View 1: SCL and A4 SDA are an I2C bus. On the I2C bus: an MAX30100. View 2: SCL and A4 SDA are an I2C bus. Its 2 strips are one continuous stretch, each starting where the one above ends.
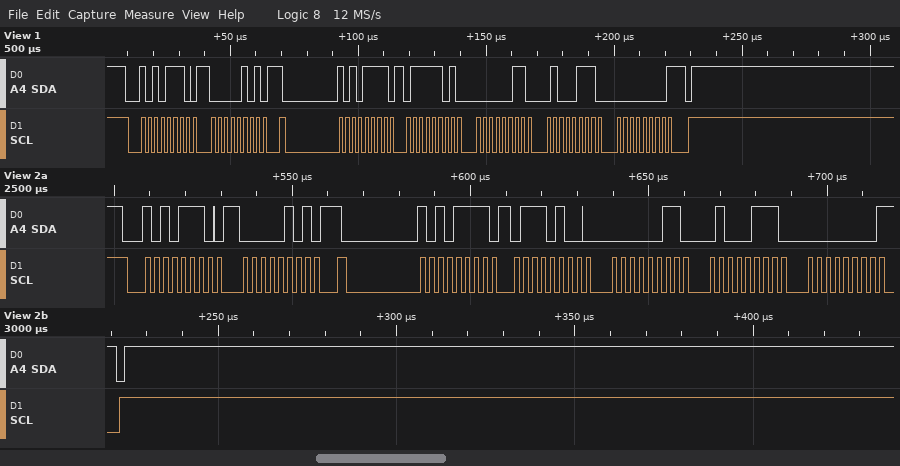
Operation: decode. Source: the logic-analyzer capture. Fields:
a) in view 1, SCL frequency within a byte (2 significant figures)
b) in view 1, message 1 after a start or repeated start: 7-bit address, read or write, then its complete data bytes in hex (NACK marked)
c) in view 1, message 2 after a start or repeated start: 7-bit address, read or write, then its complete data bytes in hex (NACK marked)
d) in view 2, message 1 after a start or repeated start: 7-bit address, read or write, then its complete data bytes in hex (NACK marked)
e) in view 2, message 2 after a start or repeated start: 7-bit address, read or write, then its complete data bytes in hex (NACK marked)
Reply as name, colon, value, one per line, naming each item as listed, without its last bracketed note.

in view 1, SCL frequency within a byte: 400 kHz
in view 1, message 1 after a start or repeated start: 7-bit address, read or write, then its complete data bytes in hex: 0x57 write: 05
in view 1, message 2 after a start or repeated start: 7-bit address, read or write, then its complete data bytes in hex: 0x57 read: 7D 03 47 00 NACK
in view 2, message 1 after a start or repeated start: 7-bit address, read or write, then its complete data bytes in hex: 0x57 write: 05
in view 2, message 2 after a start or repeated start: 7-bit address, read or write, then its complete data bytes in hex: 0x57 read: 74 03 47 00 NACK
